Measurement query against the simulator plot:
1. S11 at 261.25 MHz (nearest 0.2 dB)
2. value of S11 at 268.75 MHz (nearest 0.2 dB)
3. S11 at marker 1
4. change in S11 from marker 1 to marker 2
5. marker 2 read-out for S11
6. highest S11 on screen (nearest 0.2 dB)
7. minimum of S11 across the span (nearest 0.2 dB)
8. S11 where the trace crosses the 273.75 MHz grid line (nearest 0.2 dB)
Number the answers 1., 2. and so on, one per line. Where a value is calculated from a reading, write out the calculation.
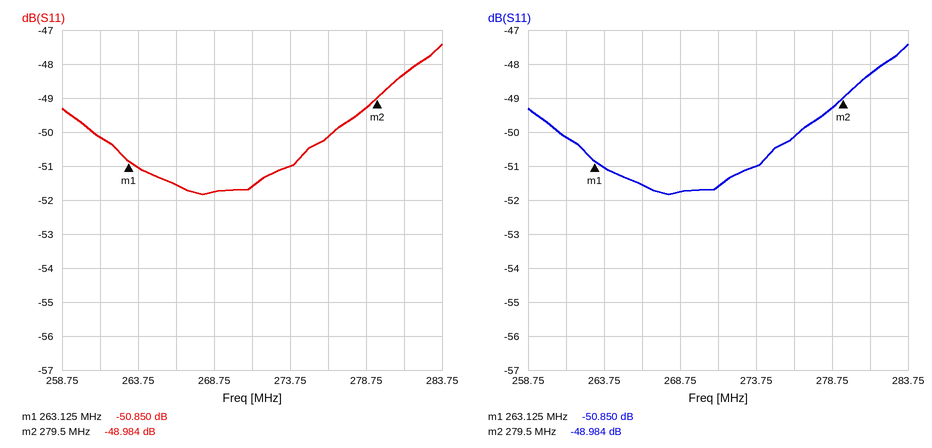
1. -50.2 dB
2. -51.8 dB
3. -50.850 dB
4. -48.984 − (-50.85) = 1.866 dB
5. -48.984 dB
6. -47.4 dB
7. -51.8 dB
8. -51.0 dB
